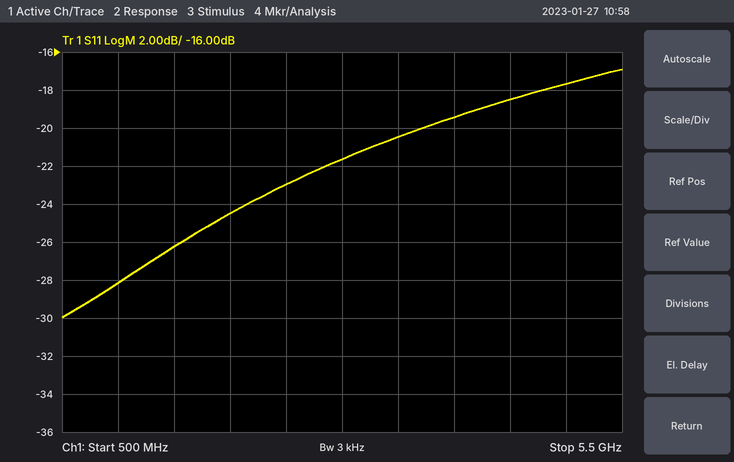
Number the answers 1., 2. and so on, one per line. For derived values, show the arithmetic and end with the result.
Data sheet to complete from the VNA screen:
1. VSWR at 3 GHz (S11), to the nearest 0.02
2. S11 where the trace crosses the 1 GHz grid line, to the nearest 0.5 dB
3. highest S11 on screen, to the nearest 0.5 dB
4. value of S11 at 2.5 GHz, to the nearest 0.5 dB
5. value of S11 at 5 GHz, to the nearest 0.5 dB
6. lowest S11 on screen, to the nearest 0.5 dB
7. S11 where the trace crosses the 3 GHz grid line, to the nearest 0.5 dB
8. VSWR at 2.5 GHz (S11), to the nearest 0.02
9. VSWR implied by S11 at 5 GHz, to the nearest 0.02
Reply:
1. |Γ| = 10^(-21.5/20) = 0.0841; VSWR = (1 + 0.0841)/(1 − 0.0841) ≈ 1.18
2. -28.0 dB
3. -17.0 dB
4. -23.0 dB
5. -17.5 dB
6. -30.0 dB
7. -21.5 dB
8. |Γ| = 10^(-23/20) = 0.0708; VSWR = (1 + 0.0708)/(1 − 0.0708) ≈ 1.15, so 1.16 to the nearest 0.02
9. |Γ| = 10^(-17.5/20) = 0.1334; VSWR = (1 + 0.1334)/(1 − 0.1334) ≈ 1.31, so 1.30 to the nearest 0.02
